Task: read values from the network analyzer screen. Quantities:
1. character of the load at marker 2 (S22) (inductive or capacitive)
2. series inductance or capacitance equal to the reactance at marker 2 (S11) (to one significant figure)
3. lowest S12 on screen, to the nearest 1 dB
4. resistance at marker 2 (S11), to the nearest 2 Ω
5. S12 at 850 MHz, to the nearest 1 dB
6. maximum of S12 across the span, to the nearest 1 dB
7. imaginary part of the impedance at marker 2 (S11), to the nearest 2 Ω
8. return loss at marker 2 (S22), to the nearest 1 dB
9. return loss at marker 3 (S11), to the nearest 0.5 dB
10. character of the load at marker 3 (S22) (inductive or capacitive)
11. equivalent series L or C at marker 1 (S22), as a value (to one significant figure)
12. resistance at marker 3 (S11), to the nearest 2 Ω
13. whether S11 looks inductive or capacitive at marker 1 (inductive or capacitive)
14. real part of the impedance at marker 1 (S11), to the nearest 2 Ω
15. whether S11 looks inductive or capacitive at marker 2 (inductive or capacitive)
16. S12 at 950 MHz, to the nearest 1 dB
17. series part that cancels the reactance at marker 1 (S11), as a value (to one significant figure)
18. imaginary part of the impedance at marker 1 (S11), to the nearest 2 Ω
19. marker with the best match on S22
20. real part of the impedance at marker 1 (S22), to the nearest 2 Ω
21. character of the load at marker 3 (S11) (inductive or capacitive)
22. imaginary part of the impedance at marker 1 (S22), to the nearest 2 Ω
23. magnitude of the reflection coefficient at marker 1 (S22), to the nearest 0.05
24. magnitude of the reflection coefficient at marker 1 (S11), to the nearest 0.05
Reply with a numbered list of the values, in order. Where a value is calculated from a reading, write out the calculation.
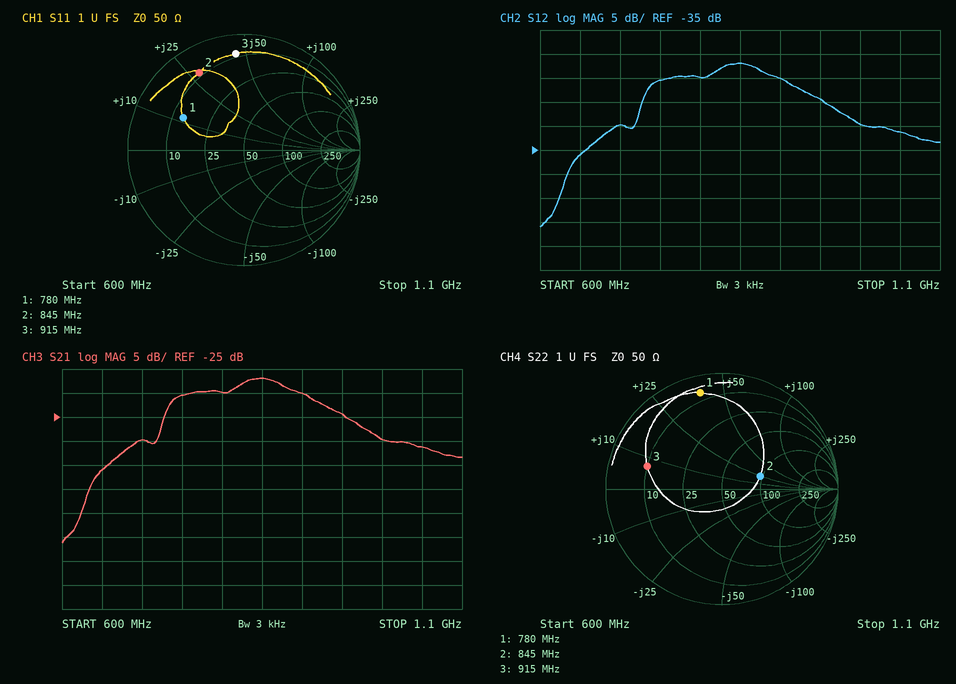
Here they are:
1. inductive
2. L = 28 Ω/(2π × 845 MHz) ≈ 5 nH
3. -51 dB
4. 8 Ω
5. -17 dB
6. -17 dB
7. +28 Ω
8. 9 dB
9. 1.5 dB
10. inductive
11. L = 40 Ω/(2π × 780 MHz) ≈ 8 nH
12. 8 Ω
13. inductive
14. 14 Ω
15. inductive
16. -24 dB
17. C = 1/(2π × 780 MHz × 12 Ω) ≈ 17.0 pF, so 20 pF to one significant figure
18. +12 Ω
19. marker 2
20. 6 Ω
21. inductive
22. +40 Ω
23. 0.85
24. 0.60
